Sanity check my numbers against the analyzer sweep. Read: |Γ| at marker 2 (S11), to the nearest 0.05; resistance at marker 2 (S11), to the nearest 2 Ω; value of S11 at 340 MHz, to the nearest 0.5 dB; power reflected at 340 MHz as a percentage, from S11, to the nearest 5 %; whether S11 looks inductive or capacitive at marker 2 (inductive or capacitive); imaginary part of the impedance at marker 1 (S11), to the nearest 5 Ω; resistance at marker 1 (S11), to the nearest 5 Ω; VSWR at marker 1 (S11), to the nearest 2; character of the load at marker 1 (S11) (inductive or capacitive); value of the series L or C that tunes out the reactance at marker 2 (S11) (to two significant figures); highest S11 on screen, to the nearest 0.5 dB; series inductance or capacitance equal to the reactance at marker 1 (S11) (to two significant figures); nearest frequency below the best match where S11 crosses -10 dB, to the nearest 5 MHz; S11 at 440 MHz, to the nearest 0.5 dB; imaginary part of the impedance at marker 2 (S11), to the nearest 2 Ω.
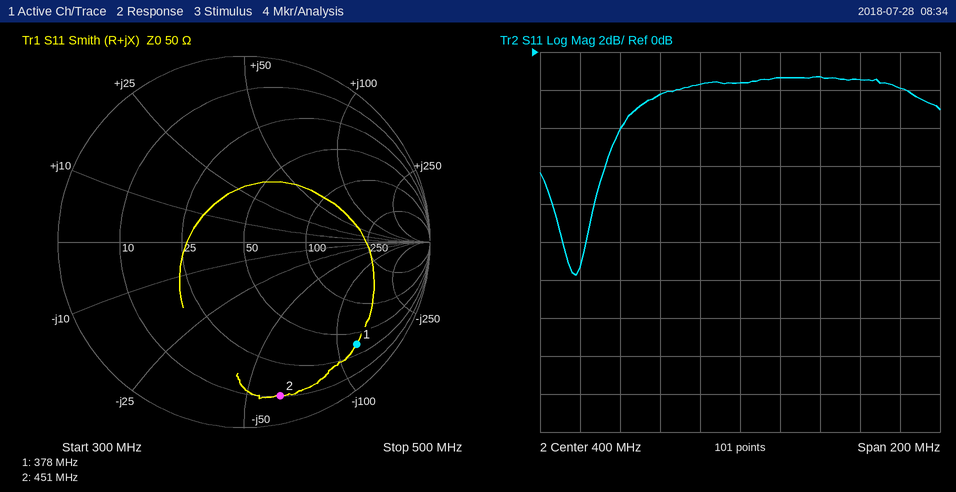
0.85
10 Ω
-4.0 dB
40 %
capacitive
-120 Ω
35 Ω
10
capacitive
22 nH
-1.5 dB
3.5 pF
310 MHz
-1.5 dB
-62 Ω
